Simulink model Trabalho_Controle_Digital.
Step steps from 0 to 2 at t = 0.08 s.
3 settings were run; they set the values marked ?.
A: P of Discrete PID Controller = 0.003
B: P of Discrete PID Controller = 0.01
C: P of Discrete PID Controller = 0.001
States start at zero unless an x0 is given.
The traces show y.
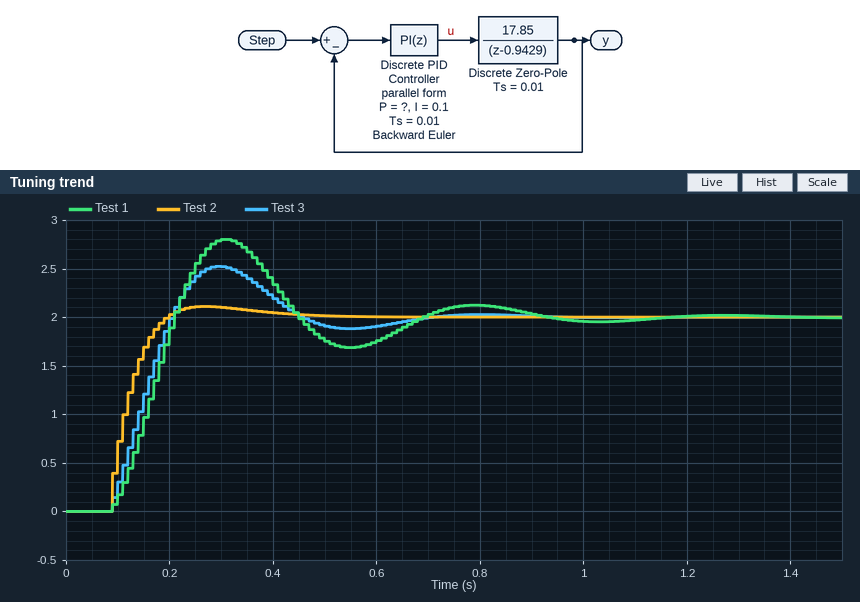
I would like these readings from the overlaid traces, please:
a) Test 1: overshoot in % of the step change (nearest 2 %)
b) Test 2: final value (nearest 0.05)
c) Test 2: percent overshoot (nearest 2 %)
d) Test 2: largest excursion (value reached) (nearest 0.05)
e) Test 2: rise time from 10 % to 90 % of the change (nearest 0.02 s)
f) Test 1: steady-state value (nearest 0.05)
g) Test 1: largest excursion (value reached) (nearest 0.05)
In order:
40 %
2.00
6 %
2.10
0.08 s
2.00
2.80
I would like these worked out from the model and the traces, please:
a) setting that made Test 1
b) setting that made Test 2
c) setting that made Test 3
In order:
C
B
A
